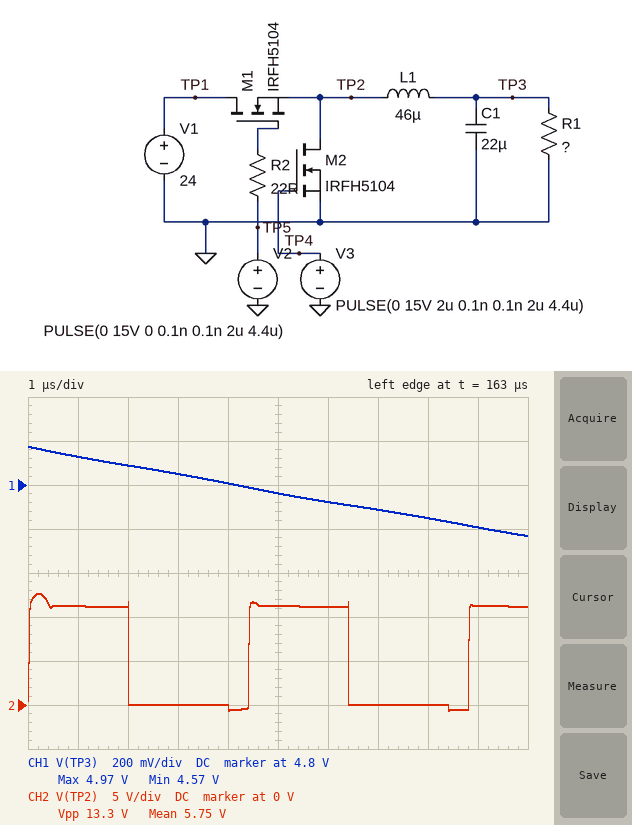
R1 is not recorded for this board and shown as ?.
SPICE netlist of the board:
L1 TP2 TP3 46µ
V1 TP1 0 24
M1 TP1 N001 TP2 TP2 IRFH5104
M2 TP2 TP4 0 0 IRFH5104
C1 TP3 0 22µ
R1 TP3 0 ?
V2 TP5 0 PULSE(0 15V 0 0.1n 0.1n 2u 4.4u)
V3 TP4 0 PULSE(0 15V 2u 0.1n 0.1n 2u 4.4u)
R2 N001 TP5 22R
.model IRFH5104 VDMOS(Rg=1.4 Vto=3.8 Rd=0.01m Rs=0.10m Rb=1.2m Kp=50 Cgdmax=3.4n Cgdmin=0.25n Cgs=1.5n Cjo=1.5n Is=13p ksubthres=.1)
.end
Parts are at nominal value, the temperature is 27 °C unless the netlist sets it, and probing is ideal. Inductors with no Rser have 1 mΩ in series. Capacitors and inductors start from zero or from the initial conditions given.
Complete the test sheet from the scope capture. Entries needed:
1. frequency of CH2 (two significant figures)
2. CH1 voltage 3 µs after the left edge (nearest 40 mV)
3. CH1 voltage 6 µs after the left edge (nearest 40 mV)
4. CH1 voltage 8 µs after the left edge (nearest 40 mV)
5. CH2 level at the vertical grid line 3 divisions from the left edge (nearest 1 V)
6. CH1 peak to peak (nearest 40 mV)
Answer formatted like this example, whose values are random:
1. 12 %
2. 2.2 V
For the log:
1. 230 kHz
2. 4.84 V
3. 4.72 V
4. 4.64 V
5. 0 V
6. 400 mV
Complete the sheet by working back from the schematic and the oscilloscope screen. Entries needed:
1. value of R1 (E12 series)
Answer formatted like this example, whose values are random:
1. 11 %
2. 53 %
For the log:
1. 4.7 Ω
